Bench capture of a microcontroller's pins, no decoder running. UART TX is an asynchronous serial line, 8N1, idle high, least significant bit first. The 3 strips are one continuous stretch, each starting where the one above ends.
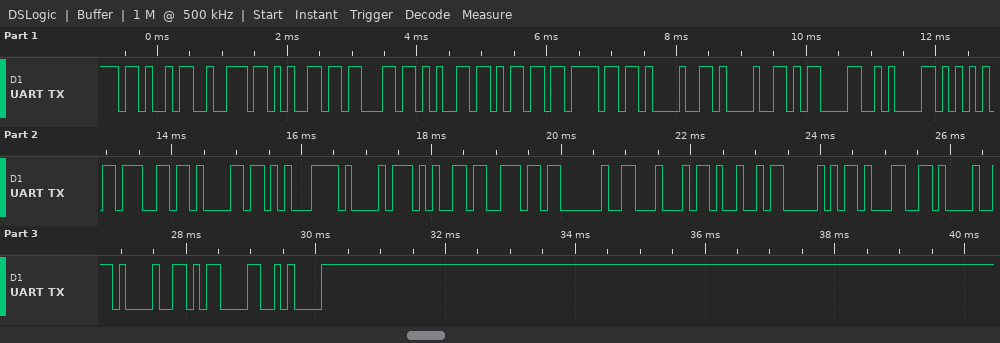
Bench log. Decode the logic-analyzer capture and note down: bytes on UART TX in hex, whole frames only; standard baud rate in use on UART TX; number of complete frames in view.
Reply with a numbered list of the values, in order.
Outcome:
1. 4B 72 65 63 65 6D 6F 21 21 0D 0A 55 67 61 C5 A1 65 6E 20 44 49 50 31 21 21 0D 0A
2. 9600 baud
3. 27
